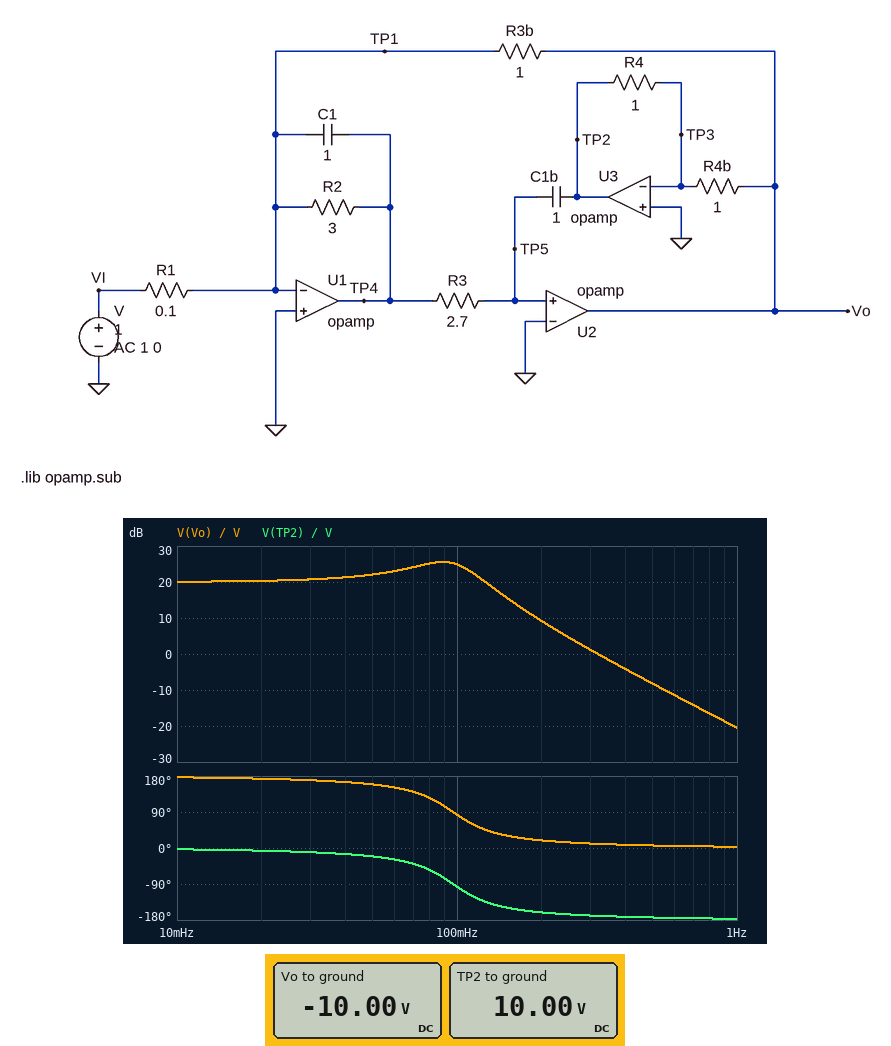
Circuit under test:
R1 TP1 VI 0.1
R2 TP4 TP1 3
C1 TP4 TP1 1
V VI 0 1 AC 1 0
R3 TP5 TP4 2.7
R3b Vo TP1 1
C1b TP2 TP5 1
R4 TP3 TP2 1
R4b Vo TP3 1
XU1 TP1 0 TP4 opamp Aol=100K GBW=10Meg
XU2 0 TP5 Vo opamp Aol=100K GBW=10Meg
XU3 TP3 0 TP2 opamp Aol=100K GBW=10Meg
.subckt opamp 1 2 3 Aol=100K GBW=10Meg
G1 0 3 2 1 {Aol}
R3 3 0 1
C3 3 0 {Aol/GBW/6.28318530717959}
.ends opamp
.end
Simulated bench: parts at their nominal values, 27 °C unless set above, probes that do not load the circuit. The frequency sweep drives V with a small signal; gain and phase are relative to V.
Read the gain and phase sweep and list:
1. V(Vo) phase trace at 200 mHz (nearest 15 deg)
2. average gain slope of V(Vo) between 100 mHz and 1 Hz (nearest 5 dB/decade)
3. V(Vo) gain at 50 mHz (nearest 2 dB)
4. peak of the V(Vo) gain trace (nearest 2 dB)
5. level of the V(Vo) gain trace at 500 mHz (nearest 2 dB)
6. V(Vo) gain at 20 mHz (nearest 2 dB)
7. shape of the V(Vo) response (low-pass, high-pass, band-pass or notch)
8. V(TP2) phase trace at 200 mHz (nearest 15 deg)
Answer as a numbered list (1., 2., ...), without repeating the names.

1. 15 deg
2. -45 dB/decade
3. 22 dB
4. 26 dB
5. -8 dB
6. 20 dB
7. low-pass
8. -165 deg
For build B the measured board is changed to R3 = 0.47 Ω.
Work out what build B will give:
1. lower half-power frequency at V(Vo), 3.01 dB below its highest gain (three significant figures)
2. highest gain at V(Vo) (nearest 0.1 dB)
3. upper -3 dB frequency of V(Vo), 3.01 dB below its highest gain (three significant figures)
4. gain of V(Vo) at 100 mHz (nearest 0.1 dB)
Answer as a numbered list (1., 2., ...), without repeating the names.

1. 201 mHz
2. 32.9 dB
3. 254 mHz
4. 21.7 dB
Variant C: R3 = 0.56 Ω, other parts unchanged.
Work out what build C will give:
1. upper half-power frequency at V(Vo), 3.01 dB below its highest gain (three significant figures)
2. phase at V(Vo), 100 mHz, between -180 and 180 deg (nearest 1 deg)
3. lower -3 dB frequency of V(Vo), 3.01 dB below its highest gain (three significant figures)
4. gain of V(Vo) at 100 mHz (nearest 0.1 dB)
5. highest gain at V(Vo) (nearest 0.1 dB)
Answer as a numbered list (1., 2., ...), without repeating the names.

1. 235 mHz
2. 171 deg
3. 181 mHz
4. 22.1 dB
5. 32.1 dB
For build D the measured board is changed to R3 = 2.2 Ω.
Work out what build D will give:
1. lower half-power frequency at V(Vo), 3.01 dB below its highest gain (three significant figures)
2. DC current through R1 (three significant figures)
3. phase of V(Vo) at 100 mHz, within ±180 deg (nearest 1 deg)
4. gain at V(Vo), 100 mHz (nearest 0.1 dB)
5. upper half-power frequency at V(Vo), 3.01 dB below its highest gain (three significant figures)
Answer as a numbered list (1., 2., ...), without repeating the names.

1. 67.7 mHz
2. 10.0 A
3. 106 deg
4. 26.4 dB
5. 125 mHz
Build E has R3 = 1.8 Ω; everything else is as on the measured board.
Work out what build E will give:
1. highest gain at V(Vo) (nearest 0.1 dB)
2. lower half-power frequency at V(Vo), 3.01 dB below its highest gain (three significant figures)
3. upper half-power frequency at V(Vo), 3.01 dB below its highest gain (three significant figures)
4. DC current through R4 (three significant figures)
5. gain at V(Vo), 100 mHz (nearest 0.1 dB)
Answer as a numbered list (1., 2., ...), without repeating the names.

1. 27.2 dB
2. 80.8 mHz
3. 137 mHz
4. 10.0 A
5. 26.5 dB
